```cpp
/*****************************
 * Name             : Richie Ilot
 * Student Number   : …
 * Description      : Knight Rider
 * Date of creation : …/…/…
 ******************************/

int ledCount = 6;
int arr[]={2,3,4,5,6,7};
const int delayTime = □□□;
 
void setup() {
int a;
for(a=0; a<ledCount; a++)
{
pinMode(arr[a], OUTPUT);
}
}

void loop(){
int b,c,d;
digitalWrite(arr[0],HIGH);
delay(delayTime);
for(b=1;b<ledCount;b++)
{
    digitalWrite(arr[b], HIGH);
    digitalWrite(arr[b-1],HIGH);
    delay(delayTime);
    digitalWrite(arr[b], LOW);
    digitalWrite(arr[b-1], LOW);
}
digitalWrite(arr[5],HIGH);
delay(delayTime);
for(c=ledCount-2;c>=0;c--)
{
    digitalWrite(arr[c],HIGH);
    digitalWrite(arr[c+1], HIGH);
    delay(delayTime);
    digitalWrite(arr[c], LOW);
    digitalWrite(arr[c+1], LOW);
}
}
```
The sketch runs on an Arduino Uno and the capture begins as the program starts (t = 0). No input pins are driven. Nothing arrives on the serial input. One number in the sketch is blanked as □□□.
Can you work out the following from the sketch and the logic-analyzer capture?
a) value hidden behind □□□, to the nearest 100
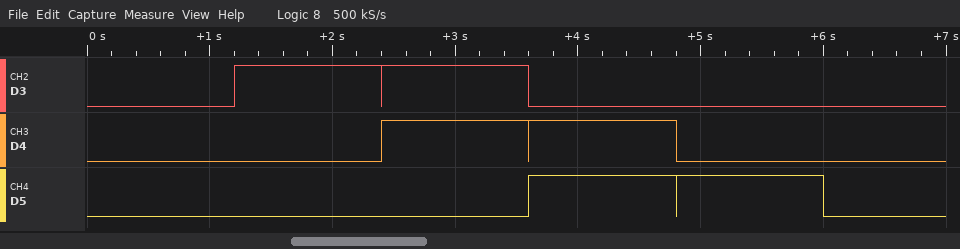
1200
